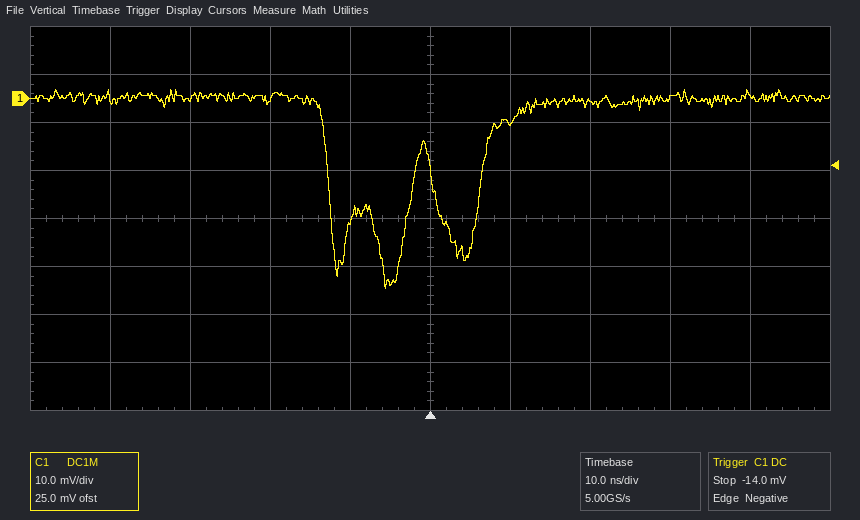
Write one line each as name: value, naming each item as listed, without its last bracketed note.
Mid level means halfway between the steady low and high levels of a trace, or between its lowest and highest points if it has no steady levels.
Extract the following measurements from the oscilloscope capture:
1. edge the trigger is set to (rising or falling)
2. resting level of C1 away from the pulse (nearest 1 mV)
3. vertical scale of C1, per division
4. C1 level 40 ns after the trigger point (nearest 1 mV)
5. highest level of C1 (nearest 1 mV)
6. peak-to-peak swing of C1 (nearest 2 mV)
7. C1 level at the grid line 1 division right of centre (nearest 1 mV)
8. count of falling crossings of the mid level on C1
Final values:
edge the trigger is set to: falling
resting level of C1 away from the pulse: 0 mV
vertical scale of C1, per division: 10 mV
C1 level 40 ns after the trigger point: 1 mV
highest level of C1: 2 mV
peak-to-peak swing of C1: 42 mV
C1 level at the grid line 1 division right of centre: -5 mV
count of falling crossings of the mid level on C1: 2
